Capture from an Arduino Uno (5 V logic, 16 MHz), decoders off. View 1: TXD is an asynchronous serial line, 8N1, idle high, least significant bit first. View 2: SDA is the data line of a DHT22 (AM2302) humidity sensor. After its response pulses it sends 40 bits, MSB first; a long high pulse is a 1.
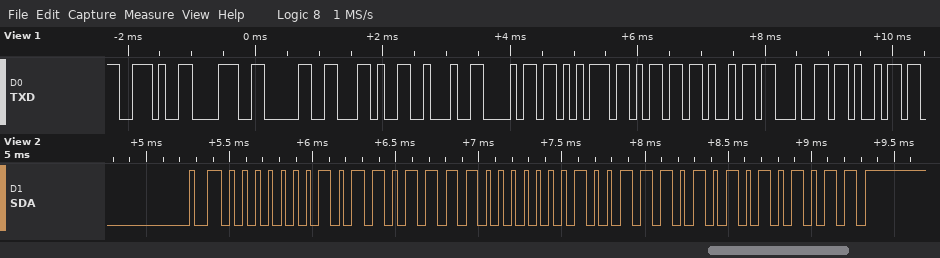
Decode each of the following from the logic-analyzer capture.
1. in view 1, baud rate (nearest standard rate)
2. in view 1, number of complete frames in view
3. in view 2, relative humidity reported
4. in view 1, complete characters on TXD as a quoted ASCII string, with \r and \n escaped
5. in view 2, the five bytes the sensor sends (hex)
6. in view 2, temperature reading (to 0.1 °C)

9600 baud
11
36.7 %
".80,\"humidi"
01 6F 01 3A AB
31.4 °C
